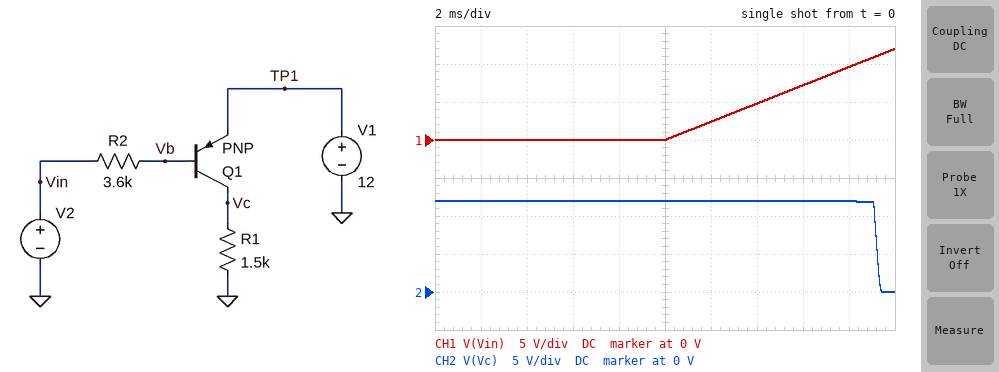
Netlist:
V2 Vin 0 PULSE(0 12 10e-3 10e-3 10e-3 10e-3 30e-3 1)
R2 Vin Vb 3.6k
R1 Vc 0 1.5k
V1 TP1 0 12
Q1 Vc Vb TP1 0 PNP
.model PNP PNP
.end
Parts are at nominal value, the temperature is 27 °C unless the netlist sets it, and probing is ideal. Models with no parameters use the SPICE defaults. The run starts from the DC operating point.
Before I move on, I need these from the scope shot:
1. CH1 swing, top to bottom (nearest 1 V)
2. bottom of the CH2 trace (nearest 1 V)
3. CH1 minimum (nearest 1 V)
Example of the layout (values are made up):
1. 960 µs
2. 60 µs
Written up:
1. 12 V
2. 0 V
3. 0 V
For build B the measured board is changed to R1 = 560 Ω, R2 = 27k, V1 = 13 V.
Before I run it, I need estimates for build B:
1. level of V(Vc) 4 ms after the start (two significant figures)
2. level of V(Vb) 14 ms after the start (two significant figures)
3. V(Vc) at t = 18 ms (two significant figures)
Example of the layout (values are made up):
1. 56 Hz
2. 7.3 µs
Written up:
1. 13 V
2. 12 V
3. 5.3 V
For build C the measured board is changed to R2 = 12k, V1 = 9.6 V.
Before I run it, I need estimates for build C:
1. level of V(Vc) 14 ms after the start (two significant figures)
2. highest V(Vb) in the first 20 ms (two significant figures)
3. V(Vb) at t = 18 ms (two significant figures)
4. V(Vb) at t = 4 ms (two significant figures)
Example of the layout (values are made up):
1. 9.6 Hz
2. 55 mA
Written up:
1. 9.5 V
2. 12 V
3. 9.6 V
4. 8.8 V
